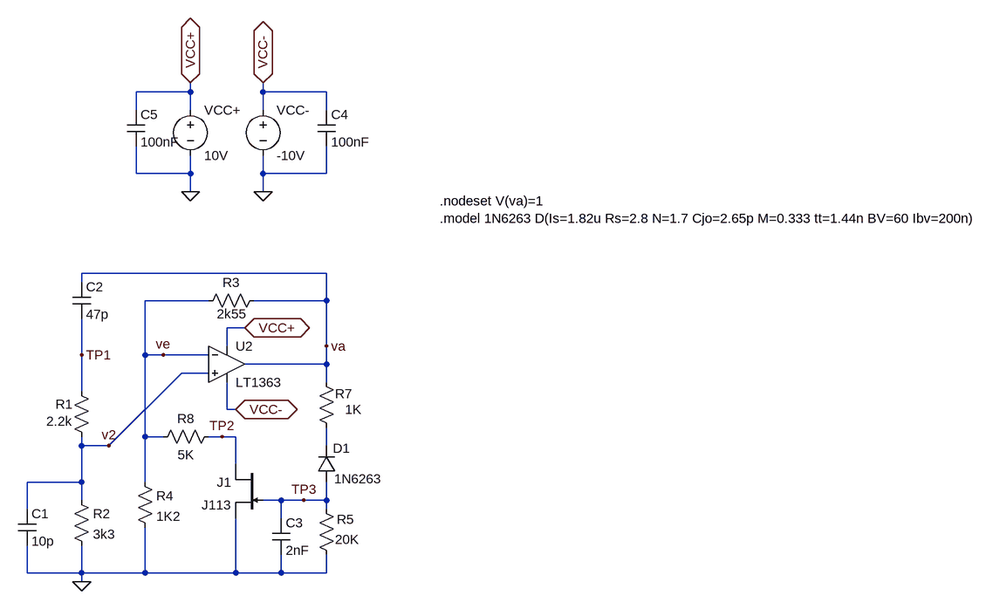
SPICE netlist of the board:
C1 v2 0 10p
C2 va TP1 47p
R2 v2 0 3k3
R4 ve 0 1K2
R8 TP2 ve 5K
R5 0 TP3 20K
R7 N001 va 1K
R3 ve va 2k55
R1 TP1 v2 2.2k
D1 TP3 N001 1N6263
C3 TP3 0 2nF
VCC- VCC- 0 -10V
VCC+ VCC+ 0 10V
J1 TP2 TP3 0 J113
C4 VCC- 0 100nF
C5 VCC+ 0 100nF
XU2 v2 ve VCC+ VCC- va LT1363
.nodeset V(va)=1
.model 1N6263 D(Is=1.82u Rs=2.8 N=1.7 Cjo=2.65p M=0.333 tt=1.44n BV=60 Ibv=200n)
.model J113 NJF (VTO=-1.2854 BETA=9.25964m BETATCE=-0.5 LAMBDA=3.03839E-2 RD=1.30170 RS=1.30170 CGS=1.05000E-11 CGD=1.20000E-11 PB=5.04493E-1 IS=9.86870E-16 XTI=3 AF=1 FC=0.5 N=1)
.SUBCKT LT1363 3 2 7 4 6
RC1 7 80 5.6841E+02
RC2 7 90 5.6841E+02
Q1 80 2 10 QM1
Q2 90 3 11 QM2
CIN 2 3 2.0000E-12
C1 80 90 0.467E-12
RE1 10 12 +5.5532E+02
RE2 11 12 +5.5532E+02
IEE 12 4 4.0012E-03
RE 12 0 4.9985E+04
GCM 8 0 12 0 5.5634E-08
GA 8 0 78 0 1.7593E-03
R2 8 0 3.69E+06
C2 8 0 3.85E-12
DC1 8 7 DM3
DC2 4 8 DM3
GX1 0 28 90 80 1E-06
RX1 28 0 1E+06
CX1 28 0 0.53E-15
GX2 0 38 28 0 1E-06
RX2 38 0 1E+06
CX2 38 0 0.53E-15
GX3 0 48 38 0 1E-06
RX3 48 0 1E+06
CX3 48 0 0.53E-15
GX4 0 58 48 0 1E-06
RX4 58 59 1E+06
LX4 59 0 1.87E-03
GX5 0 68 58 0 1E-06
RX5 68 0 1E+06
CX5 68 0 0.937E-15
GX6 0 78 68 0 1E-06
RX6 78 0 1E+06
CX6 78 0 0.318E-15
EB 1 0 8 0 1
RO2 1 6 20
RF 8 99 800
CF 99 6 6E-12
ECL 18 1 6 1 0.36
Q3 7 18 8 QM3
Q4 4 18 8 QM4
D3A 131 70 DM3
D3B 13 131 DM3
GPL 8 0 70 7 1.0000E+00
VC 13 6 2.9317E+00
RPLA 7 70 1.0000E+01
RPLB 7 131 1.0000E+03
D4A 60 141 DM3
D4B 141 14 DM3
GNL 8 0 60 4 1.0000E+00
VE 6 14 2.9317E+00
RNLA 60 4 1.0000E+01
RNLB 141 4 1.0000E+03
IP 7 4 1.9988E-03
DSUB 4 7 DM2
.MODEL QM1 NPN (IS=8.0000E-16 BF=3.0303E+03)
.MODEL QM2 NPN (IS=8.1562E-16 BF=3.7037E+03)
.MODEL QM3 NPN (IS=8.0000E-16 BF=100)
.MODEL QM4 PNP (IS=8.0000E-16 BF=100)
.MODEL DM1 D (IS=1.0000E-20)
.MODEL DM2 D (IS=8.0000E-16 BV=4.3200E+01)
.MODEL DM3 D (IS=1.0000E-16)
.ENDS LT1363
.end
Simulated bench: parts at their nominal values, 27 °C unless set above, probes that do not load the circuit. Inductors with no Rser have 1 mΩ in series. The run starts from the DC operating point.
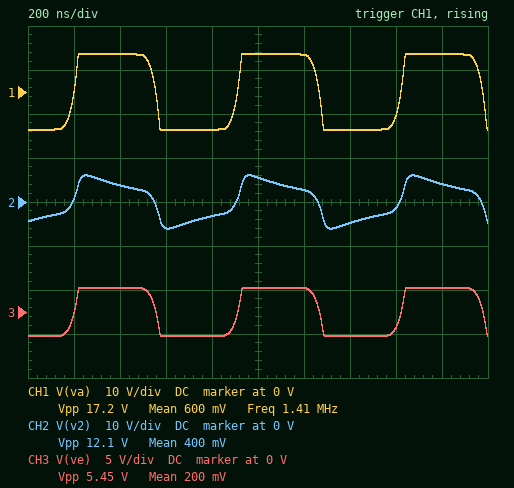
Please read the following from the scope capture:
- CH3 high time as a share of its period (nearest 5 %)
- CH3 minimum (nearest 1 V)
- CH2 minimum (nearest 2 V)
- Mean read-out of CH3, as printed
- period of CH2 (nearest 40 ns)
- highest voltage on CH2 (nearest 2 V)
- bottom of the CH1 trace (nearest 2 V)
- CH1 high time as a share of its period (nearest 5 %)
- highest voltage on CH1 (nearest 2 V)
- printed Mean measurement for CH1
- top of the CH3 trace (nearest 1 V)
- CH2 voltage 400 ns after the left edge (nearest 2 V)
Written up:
50 %
-3 V
-6 V
200 mV
720 ns
6 V
-8 V
50 %
8 V
600 mV
3 V
4 V
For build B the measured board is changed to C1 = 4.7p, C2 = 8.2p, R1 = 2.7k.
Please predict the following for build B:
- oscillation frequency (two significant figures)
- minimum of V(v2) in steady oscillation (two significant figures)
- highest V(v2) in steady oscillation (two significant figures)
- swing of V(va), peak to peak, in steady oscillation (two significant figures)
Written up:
5.1 MHz
-4.3 V
4.3 V
17 V
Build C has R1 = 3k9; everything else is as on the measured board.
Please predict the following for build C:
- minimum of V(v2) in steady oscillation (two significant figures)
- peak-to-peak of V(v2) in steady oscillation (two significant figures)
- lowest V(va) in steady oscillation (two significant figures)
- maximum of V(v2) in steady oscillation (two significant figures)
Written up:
-4.4 V
8.7 V
-8.6 V
4.4 V
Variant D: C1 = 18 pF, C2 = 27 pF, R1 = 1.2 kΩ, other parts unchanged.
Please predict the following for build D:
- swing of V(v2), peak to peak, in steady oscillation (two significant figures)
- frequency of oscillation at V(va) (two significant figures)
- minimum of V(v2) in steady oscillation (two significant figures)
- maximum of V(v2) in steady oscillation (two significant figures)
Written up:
11 V
2.2 MHz
-5.4 V
5.4 V
